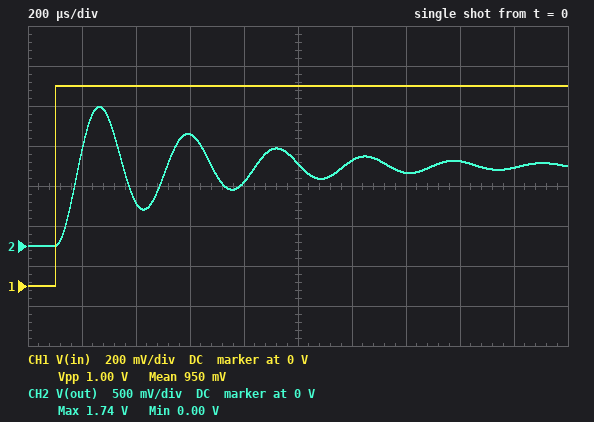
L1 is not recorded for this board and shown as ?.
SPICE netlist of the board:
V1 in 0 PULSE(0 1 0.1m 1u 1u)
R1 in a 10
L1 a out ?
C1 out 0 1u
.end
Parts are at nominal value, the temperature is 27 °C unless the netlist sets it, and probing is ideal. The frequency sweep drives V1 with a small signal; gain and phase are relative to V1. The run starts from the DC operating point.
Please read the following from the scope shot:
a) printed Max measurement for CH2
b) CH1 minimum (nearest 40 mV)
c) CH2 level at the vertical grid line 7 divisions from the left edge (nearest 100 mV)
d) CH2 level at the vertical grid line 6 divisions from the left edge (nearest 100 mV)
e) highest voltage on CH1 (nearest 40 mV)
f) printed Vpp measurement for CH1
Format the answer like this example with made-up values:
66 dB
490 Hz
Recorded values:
1.74 V
0 V
900 mV
1.1 V
1.00 V
1.00 V
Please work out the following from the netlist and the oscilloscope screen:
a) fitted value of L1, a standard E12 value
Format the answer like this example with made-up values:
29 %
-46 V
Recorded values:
2.7 mH
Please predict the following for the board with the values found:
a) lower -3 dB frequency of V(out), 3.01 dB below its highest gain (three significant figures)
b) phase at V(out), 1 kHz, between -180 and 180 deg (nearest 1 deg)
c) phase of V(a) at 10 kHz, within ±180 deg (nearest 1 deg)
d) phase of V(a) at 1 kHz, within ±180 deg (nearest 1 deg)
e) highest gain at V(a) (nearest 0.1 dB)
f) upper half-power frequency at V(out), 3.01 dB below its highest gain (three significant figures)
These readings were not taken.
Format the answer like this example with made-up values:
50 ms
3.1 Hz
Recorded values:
2.72 kHz
-4 deg
4 deg
-4 deg
0 dB
3.32 kHz
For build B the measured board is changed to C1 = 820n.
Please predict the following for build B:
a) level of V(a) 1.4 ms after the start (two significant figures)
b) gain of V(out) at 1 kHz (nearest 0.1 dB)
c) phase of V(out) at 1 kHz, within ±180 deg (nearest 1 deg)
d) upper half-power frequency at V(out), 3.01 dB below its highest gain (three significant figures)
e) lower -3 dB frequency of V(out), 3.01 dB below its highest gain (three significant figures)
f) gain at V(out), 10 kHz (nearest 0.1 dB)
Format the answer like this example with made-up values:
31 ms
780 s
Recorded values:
990 mV
0.8 dB
-3 deg
3.64 kHz
3.05 kHz
-17.8 dB
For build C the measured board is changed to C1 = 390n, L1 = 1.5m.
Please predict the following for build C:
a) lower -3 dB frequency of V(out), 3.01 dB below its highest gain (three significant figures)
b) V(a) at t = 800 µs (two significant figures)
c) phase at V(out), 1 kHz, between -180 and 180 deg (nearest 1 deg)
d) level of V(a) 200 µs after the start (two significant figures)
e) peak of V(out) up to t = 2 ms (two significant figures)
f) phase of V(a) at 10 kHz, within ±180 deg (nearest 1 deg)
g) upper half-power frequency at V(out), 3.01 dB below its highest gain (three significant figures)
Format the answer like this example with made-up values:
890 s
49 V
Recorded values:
5.98 kHz
1.0 V
-1 deg
1.1 V
1.8 V
11 deg
7.05 kHz
